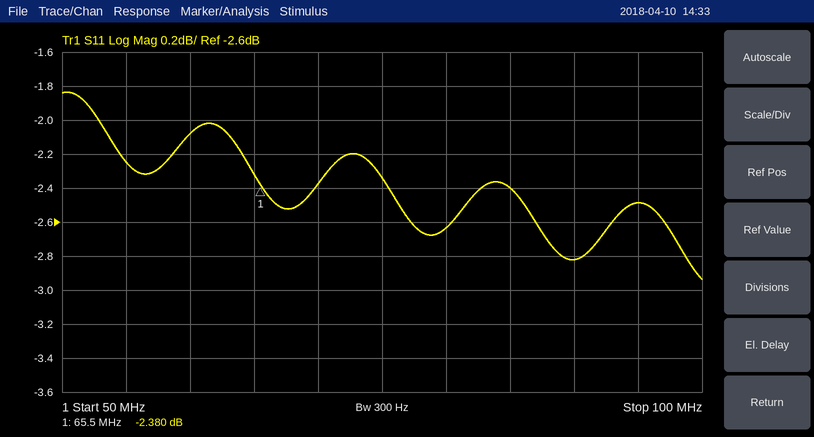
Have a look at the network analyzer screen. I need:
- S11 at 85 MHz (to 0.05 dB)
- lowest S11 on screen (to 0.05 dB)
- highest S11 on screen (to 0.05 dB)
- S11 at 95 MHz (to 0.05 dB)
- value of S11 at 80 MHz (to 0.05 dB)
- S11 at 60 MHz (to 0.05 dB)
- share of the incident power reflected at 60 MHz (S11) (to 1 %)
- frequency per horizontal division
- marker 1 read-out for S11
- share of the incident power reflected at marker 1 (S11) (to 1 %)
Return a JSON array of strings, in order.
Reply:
["-2.40 dB", "-2.95 dB", "-1.85 dB", "-2.50 dB", "-2.65 dB", "-2.10 dB", "62 %", "5 MHz", "-2.380 dB", "58 %"]
